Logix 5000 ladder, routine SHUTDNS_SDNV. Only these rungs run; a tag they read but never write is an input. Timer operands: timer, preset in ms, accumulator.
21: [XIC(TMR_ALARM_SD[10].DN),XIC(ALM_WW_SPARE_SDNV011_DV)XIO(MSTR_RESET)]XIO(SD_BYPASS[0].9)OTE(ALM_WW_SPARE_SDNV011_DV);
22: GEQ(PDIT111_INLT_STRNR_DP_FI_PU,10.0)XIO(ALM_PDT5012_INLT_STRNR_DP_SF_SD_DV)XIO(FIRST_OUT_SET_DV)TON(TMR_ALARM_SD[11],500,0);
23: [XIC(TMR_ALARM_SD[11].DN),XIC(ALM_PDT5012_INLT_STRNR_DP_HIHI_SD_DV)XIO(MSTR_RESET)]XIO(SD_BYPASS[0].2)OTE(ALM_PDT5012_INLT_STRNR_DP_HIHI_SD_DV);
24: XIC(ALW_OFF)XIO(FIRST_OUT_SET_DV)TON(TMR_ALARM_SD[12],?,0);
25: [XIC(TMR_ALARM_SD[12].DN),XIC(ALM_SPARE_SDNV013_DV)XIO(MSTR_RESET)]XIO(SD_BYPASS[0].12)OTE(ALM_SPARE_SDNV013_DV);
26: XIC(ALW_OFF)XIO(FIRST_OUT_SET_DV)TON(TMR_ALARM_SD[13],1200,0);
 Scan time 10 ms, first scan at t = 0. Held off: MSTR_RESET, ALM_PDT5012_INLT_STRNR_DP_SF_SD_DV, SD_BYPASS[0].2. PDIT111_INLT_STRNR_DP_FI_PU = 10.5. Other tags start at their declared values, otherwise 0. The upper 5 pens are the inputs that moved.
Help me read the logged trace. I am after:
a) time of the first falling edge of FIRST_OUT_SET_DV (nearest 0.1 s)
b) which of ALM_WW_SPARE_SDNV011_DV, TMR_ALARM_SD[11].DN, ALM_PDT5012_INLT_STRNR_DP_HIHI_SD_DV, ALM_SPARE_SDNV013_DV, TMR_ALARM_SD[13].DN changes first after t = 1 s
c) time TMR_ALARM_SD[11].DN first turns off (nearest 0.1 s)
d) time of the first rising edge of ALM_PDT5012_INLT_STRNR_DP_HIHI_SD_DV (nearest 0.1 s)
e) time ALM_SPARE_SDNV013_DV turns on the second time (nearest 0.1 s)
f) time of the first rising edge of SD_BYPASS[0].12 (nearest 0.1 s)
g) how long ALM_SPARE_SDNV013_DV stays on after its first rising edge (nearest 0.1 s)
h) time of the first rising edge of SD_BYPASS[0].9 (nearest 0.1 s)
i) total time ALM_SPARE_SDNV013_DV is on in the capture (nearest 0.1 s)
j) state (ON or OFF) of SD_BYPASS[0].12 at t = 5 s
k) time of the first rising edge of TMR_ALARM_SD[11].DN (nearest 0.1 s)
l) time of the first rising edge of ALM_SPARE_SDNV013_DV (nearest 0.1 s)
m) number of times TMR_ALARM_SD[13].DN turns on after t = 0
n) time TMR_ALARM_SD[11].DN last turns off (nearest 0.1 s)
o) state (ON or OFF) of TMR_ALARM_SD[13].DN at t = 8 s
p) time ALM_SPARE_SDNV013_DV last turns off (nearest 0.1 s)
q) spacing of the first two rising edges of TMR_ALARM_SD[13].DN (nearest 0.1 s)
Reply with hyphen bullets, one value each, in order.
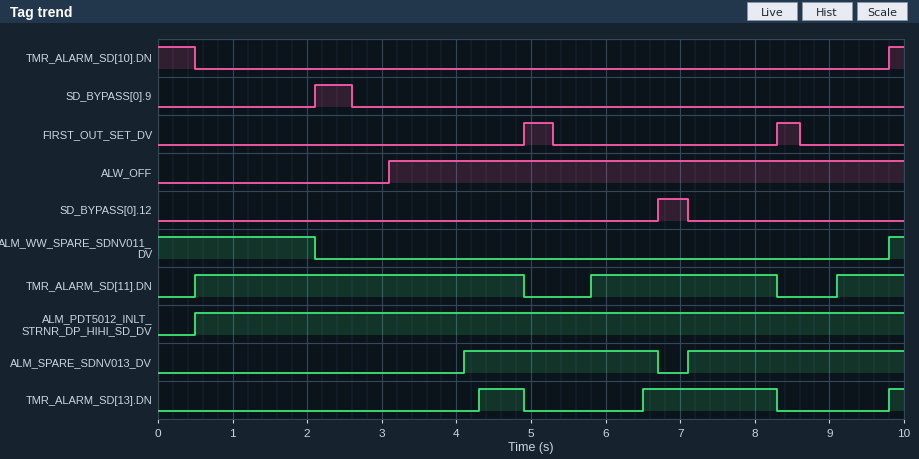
- 5.3 s
- ALM_WW_SPARE_SDNV011_DV
- 4.9 s
- 0.5 s
- 7.1 s
- 6.7 s
- 2.6 s
- 2.1 s
- 5.5 s
- OFF
- 0.5 s
- 4.1 s
- 3
- 8.3 s
- ON
- 6.7 s
- 2.2 s
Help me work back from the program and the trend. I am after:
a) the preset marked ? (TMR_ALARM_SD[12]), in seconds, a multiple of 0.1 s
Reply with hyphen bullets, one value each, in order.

- 1.0 s
